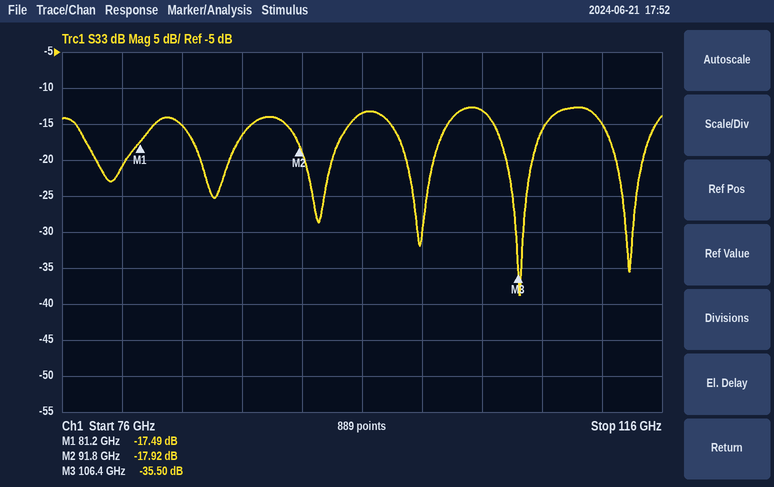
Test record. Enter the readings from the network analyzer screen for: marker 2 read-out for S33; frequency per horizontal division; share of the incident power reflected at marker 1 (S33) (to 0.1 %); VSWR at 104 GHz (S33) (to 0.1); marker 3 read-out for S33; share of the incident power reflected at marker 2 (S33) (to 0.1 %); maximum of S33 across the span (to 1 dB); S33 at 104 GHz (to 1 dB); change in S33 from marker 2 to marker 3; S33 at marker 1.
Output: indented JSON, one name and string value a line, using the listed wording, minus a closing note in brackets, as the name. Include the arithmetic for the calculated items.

{
  "marker 2 read-out for S33": "-17.92 dB",
  "frequency per horizontal division": "4 GHz",
  "share of the incident power reflected at marker 1 (S33)": "10^(-17.49/10) ≈ 1.8 %",
  "VSWR at 104 GHz (S33)": "|Γ| = 10^(-13/20) = 0.2239; VSWR = (1 + 0.2239)/(1 − 0.2239) ≈ 1.6",
  "marker 3 read-out for S33": "-35.50 dB",
  "share of the incident power reflected at marker 2 (S33)": "10^(-17.92/10) ≈ 1.6 %",
  "maximum of S33 across the span": "-13 dB",
  "S33 at 104 GHz": "-13 dB",
  "change in S33 from marker 2 to marker 3": "-35.5 − (-17.92) = -17.58 dB",
  "S33 at marker 1": "-17.49 dB"
}
